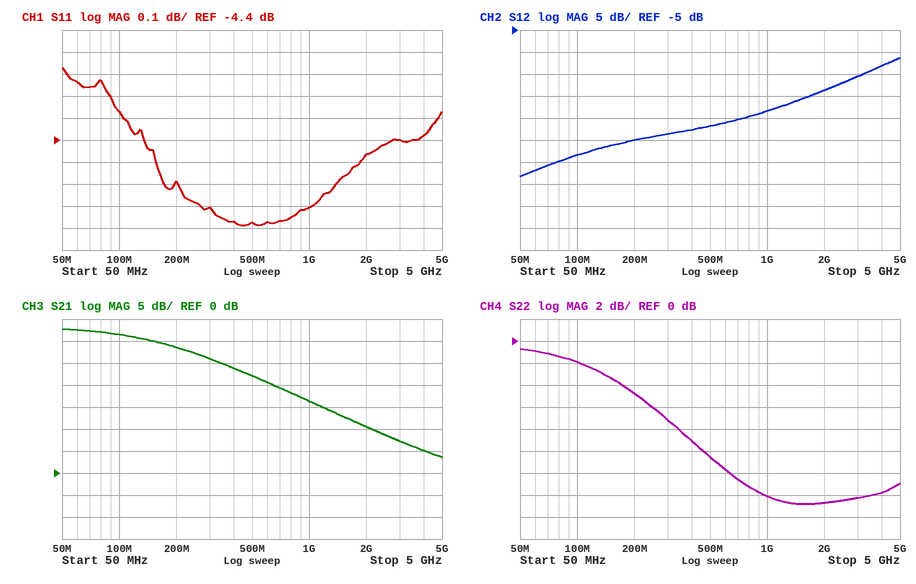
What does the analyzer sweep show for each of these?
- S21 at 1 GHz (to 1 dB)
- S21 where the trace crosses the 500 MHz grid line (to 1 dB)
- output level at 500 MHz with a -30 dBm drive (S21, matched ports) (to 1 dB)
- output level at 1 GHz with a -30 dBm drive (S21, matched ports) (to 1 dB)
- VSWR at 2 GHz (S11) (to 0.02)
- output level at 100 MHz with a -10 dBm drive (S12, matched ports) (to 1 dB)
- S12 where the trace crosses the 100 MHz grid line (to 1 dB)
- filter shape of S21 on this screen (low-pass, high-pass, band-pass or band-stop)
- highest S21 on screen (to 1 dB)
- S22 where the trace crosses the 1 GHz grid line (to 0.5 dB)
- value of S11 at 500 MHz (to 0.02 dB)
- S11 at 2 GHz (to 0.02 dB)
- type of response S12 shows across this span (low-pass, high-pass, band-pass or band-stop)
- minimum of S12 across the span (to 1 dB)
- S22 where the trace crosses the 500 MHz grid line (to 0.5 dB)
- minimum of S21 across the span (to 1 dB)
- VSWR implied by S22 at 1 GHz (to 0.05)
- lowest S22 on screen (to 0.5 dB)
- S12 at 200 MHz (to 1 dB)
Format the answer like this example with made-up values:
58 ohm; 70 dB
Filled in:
16 dB; 22 dB; -8 dBm; -14 dBm; 3.98; -43 dBm; -33 dB; low-pass; 33 dB; -14.0 dB; -4.78 dB; -4.46 dB; high-pass; -38 dB; -10.5 dB; 4 dB; 1.50; -15.0 dB; -30 dB
